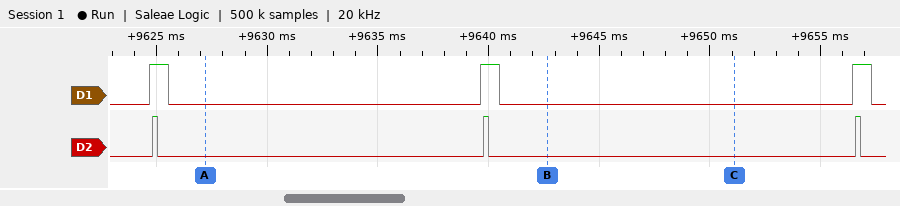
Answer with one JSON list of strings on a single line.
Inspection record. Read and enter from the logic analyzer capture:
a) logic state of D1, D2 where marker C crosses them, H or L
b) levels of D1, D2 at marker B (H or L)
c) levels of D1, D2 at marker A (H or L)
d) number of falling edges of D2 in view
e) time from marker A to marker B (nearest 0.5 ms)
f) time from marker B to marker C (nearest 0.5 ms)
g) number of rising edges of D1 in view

["D1=L, D2=L", "D1=L, D2=L", "D1=L, D2=L", "3", "15.5 ms", "8.5 ms", "3"]
